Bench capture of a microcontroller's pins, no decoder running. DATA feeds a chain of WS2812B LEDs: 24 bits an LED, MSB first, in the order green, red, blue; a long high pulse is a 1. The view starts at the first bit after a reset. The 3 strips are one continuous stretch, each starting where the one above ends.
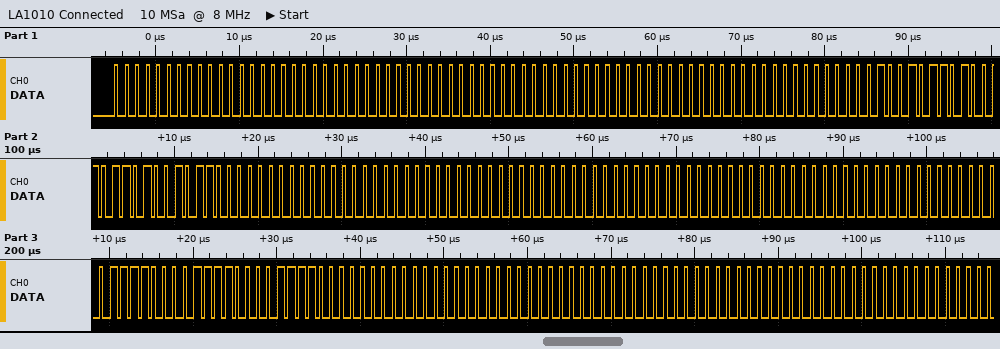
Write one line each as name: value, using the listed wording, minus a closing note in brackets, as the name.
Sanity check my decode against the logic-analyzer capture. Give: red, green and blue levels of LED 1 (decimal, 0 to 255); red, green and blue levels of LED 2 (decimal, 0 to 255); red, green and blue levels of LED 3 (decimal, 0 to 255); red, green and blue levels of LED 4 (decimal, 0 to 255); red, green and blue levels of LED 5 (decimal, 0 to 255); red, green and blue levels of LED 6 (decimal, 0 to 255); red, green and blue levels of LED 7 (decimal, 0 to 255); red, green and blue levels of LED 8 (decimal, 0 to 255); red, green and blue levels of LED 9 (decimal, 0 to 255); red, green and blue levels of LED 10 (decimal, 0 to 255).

red, green and blue levels of LED 1: 0, 0, 0
red, green and blue levels of LED 2: 0, 0, 0
red, green and blue levels of LED 3: 0, 0, 0
red, green and blue levels of LED 4: 75, 75, 75
red, green and blue levels of LED 5: 0, 0, 0
red, green and blue levels of LED 6: 0, 0, 0
red, green and blue levels of LED 7: 0, 0, 0
red, green and blue levels of LED 8: 15, 15, 15
red, green and blue levels of LED 9: 0, 0, 0
red, green and blue levels of LED 10: 0, 0, 0
